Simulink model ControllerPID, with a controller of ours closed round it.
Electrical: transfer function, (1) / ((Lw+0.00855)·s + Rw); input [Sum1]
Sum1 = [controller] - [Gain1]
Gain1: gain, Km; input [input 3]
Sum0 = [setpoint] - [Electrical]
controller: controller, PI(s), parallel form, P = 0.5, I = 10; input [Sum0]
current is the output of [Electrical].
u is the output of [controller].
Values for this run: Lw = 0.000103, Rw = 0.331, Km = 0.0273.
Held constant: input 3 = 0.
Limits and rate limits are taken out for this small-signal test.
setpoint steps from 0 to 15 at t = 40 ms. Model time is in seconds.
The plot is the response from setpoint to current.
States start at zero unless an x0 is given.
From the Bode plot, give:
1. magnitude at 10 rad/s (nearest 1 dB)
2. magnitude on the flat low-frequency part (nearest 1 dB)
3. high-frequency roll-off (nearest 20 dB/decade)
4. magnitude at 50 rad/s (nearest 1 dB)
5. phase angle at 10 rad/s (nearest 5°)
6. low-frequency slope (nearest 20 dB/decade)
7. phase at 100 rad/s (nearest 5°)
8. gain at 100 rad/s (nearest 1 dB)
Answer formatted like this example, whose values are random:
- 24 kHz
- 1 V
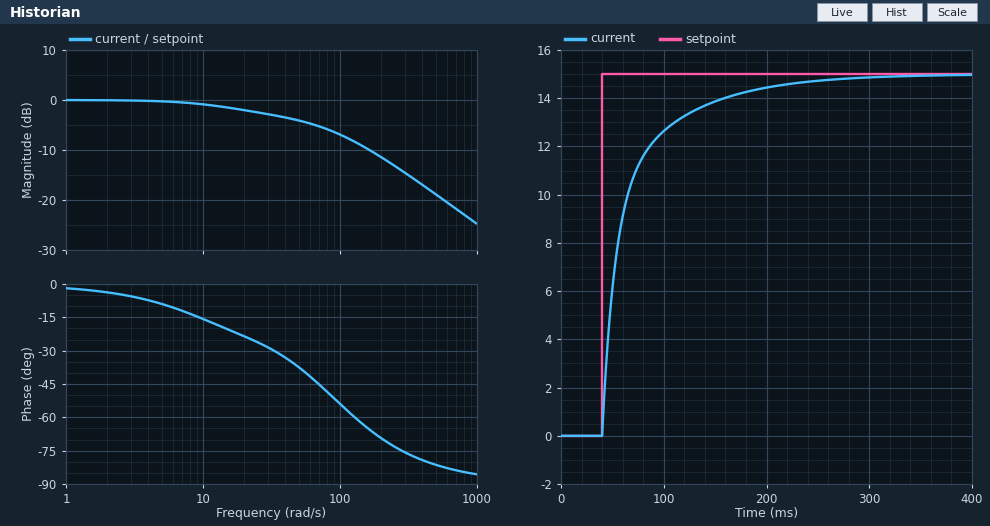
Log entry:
- -1 dB
- 0 dB
- -20 dB/decade
- -4 dB
- -15°
- 0 dB/decade
- -55°
- -7 dB
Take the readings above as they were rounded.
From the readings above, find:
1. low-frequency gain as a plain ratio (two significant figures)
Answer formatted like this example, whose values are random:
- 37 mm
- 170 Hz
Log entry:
- 1.0
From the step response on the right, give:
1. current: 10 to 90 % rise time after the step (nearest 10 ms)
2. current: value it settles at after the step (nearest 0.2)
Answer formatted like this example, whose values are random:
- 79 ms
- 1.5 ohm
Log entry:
- 90 ms
- 15.0
